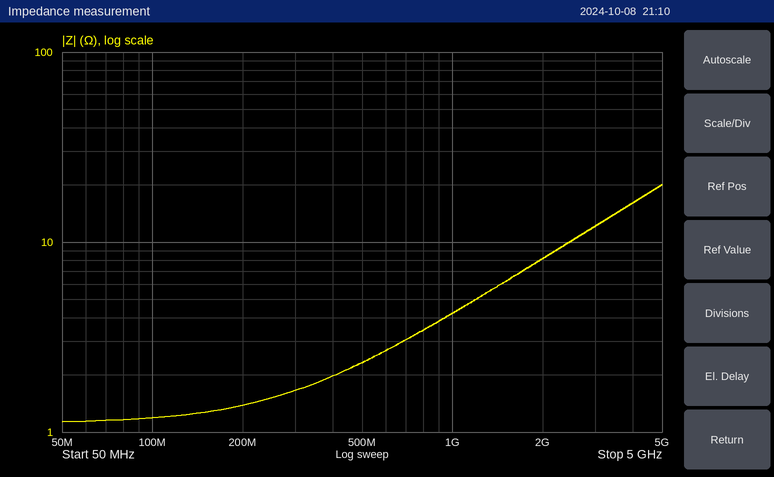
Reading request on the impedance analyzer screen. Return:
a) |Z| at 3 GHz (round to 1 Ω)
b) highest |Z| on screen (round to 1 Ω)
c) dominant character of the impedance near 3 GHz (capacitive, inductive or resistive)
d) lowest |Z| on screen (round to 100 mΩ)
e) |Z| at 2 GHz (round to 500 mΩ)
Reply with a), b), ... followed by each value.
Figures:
a) 12 Ω
b) 20 Ω
c) inductive
d) 1.1 Ω
e) 8.0 Ω
